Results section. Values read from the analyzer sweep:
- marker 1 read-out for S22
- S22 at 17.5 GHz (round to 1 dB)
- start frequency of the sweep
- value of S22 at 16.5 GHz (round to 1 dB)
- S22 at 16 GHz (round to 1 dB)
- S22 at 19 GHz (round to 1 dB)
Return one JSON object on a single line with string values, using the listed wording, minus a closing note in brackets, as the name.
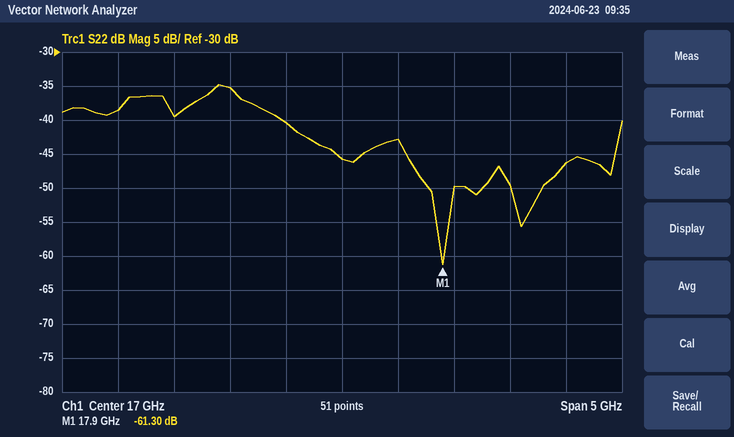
{"marker 1 read-out for S22": "-61.30 dB", "S22 at 17.5 GHz": "-43 dB", "start frequency of the sweep": "14.5 GHz", "value of S22 at 16.5 GHz": "-40 dB", "S22 at 16 GHz": "-35 dB", "S22 at 19 GHz": "-46 dB"}
